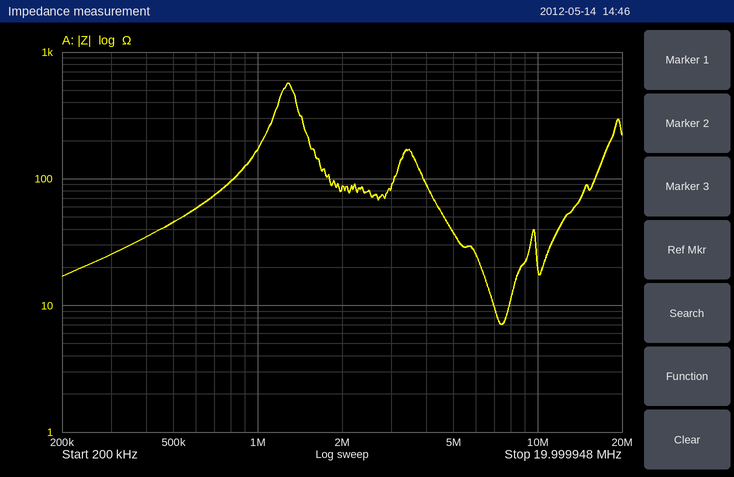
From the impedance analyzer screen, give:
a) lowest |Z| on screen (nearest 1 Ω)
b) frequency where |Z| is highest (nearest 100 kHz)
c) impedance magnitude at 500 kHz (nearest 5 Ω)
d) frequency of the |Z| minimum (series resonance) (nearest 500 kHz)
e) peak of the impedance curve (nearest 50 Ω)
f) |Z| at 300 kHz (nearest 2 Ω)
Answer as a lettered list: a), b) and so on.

a) 7 Ω
b) 1.3 MHz
c) 45 Ω
d) 7.5 MHz
e) 550 Ω
f) 26 Ω
